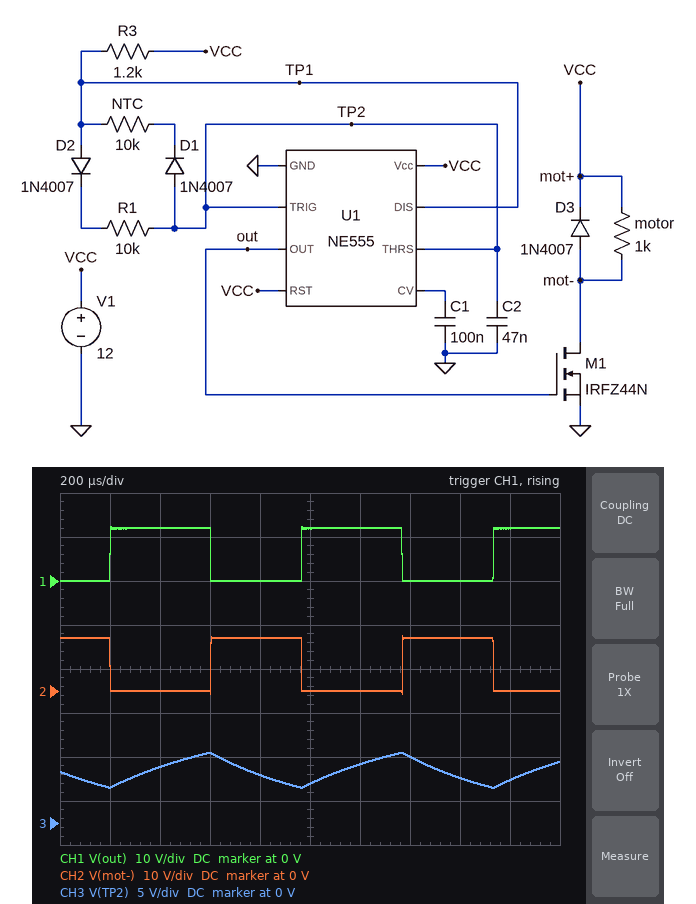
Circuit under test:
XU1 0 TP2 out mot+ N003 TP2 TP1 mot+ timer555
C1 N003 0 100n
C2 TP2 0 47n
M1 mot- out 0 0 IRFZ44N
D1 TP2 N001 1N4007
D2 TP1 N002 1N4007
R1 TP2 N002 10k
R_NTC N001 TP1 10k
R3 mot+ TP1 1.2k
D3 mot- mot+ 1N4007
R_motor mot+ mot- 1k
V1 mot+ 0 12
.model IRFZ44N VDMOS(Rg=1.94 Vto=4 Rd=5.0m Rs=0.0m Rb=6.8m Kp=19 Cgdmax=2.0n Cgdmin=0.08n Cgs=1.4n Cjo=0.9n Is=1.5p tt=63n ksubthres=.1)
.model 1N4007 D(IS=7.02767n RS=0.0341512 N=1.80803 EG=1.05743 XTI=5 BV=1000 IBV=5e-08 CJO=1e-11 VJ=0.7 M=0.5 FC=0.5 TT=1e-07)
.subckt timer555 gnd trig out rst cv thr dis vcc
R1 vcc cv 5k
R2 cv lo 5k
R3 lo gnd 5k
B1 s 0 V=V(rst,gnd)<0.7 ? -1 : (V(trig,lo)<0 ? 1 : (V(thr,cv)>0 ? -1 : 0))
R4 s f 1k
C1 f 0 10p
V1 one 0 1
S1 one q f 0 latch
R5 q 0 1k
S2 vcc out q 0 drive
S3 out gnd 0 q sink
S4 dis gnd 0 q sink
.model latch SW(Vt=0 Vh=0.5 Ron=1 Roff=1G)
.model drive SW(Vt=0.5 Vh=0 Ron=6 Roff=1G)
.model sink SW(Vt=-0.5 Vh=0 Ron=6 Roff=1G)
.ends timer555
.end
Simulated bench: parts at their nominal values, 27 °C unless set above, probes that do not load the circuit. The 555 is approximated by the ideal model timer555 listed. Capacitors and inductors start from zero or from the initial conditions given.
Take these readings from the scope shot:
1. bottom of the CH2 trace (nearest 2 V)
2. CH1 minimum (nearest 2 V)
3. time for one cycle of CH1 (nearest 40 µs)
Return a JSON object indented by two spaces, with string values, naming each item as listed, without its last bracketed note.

{
  "bottom of the CH2 trace": "0 V",
  "CH1 minimum": "0 V",
  "time for one cycle of CH1": "760 µs"
}
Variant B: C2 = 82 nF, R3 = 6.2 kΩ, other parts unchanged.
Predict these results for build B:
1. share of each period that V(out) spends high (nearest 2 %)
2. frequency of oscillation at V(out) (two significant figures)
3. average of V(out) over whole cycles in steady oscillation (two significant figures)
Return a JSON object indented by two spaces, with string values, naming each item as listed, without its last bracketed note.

{
  "share of each period that V(out) spends high": "62 %",
  "frequency of oscillation at V(out)": "610 Hz",
  "average of V(out) over whole cycles in steady oscillation": "7.4 V"
}
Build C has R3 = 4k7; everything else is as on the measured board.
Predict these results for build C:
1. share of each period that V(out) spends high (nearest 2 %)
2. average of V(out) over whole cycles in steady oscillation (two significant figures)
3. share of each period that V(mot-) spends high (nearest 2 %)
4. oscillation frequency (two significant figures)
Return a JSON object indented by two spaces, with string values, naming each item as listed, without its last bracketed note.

{
  "share of each period that V(out) spends high": "60 %",
  "average of V(out) over whole cycles in steady oscillation": "7.1 V",
  "share of each period that V(mot-) spends high": "40 %",
  "oscillation frequency": "1.1 kHz"
}
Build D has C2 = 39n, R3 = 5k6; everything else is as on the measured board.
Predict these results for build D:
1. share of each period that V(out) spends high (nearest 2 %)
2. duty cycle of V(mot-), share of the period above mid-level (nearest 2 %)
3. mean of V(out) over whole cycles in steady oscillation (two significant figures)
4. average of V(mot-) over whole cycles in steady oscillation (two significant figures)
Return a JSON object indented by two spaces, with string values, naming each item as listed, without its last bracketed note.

{
  "share of each period that V(out) spends high": "60 %",
  "duty cycle of V(mot-), share of the period above mid-level": "40 %",
  "mean of V(out) over whole cycles in steady oscillation": "7.3 V",
  "average of V(mot-) over whole cycles in steady oscillation": "4.7 V"
}
